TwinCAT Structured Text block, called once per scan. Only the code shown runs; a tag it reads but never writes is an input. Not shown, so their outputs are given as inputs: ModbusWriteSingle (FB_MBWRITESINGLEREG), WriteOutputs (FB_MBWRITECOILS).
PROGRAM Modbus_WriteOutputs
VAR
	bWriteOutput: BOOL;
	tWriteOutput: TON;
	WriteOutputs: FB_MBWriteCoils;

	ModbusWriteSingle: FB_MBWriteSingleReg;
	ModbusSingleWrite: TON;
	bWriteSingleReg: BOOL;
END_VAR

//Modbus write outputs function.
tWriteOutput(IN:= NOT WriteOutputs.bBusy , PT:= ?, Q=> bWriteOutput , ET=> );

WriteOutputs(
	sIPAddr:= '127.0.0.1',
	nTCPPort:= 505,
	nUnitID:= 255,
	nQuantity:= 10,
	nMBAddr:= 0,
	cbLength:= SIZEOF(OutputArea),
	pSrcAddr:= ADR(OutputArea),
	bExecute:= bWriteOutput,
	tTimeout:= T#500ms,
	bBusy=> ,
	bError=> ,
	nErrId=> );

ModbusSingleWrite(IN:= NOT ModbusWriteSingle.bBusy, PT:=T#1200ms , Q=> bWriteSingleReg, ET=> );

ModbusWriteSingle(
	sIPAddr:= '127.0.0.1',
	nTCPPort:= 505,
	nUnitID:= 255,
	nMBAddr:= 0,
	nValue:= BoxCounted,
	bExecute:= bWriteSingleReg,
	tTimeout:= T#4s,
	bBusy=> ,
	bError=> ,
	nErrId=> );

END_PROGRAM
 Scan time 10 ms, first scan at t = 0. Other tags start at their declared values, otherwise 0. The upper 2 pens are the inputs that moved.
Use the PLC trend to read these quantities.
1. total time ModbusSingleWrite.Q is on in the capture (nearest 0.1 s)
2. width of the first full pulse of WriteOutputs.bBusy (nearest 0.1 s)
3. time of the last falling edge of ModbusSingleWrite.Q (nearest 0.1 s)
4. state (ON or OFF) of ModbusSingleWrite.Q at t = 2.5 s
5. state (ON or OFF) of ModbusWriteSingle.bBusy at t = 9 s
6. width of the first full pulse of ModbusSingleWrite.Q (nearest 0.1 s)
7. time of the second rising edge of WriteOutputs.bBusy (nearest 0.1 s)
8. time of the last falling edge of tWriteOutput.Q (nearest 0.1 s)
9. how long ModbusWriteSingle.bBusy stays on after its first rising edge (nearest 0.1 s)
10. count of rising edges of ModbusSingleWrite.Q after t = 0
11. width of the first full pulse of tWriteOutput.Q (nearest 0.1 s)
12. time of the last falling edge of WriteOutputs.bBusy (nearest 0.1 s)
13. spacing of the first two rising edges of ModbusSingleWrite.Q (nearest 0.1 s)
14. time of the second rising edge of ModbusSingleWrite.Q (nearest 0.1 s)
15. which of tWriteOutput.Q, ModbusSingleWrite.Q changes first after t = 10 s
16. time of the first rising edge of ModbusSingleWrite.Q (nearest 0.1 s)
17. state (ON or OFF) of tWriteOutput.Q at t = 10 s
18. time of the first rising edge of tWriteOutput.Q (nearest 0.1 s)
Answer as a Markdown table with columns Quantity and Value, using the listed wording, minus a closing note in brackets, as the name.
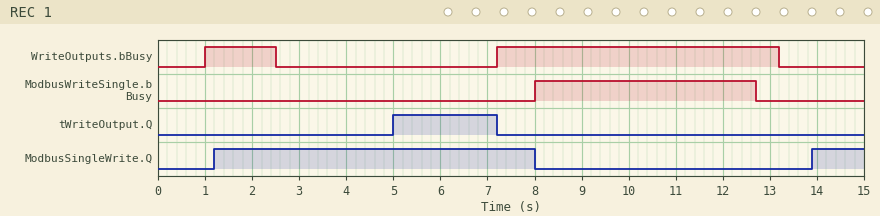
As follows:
| Quantity | Value |
|---|---|
| total time ModbusSingleWrite.Q is on in the capture | 7.9 s |
| width of the first full pulse of WriteOutputs.bBusy | 1.5 s |
| time of the last falling edge of ModbusSingleWrite.Q | 8.0 s |
| state (ON or OFF) of ModbusSingleWrite.Q at t = 2.5 s | ON |
| state (ON or OFF) of ModbusWriteSingle.bBusy at t = 9 s | ON |
| width of the first full pulse of ModbusSingleWrite.Q | 6.8 s |
| time of the second rising edge of WriteOutputs.bBusy | 7.2 s |
| time of the last falling edge of tWriteOutput.Q | 7.2 s |
| how long ModbusWriteSingle.bBusy stays on after its first rising edge | 4.7 s |
| count of rising edges of ModbusSingleWrite.Q after t = 0 | 2 |
| width of the first full pulse of tWriteOutput.Q | 2.2 s |
| time of the last falling edge of WriteOutputs.bBusy | 13.2 s |
| spacing of the first two rising edges of ModbusSingleWrite.Q | 12.7 s |
| time of the second rising edge of ModbusSingleWrite.Q | 13.9 s |
| which of tWriteOutput.Q, ModbusSingleWrite.Q changes first after t = 10 s | ModbusSingleWrite.Q |
| time of the first rising edge of ModbusSingleWrite.Q | 1.2 s |
| state (ON or OFF) of tWriteOutput.Q at t = 10 s | OFF |
| time of the first rising edge of tWriteOutput.Q | 5.0 s |
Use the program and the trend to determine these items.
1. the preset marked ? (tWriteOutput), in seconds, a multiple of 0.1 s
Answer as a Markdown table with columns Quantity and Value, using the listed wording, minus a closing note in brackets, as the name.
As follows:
| Quantity | Value |
|---|---|
| the preset marked ? (tWriteOutput), in seconds, a multiple of 0.1 s | 2.5 s |
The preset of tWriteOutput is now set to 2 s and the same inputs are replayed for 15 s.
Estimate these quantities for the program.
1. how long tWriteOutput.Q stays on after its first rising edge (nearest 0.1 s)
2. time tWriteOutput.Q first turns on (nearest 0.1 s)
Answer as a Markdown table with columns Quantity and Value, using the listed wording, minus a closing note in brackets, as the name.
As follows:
| Quantity | Value |
|---|---|
| how long tWriteOutput.Q stays on after its first rising edge | 2.7 s |
| time tWriteOutput.Q first turns on | 4.5 s |
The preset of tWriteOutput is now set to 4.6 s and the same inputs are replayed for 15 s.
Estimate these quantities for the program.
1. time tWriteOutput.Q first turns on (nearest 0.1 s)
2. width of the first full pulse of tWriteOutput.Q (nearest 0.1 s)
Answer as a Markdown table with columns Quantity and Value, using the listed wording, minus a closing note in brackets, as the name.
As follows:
| Quantity | Value |
|---|---|
| time tWriteOutput.Q first turns on | 7.1 s |
| width of the first full pulse of tWriteOutput.Q | 0.1 s |
